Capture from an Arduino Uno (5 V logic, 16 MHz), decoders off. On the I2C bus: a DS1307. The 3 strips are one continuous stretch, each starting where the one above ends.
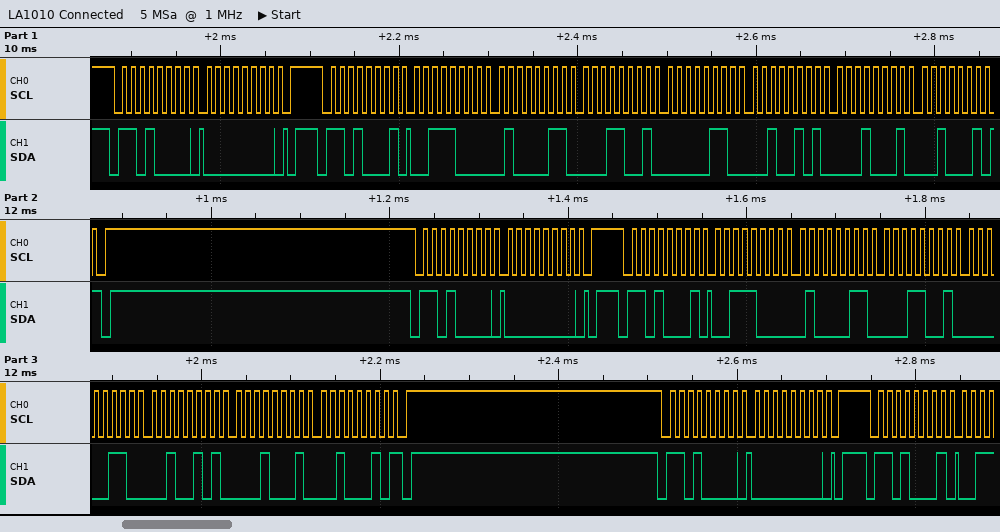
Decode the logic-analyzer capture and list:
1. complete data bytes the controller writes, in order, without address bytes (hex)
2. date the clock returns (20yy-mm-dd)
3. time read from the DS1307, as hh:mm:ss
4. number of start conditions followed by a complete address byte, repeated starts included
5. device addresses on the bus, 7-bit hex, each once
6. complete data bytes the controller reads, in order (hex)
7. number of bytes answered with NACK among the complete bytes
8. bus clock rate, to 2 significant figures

00 00 00
2022-11-25
19:43:38
6
0x68
38 43 19 06 25 11 22 38 43 19 06 25 11 22
2
100 kHz
